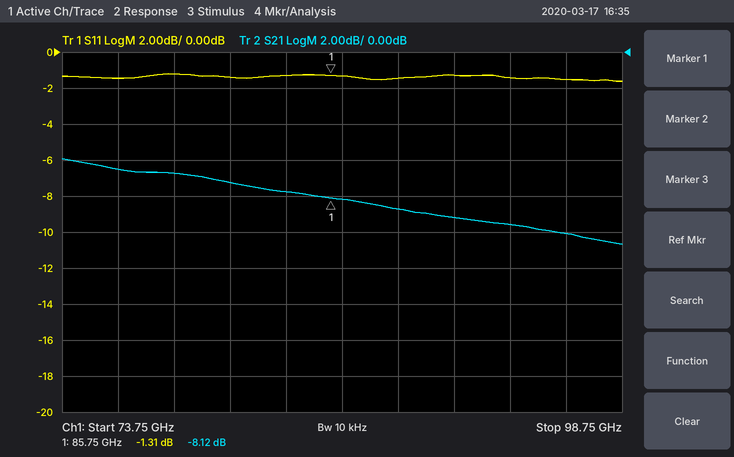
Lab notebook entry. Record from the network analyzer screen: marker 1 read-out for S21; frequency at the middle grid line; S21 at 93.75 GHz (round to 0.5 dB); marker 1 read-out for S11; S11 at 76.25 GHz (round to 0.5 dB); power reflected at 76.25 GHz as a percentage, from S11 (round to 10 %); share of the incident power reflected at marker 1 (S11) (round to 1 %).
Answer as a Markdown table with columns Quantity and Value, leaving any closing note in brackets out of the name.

| Quantity | Value |
|---|---|
| marker 1 read-out for S21 | -8.12 dB |
| frequency at the middle grid line | 86.25 GHz |
| S21 at 93.75 GHz | -9.5 dB |
| marker 1 read-out for S11 | -1.31 dB |
| S11 at 76.25 GHz | -1.5 dB |
| power reflected at 76.25 GHz as a percentage, from S11 | 70 % |
| share of the incident power reflected at marker 1 (S11) | 74 % |
